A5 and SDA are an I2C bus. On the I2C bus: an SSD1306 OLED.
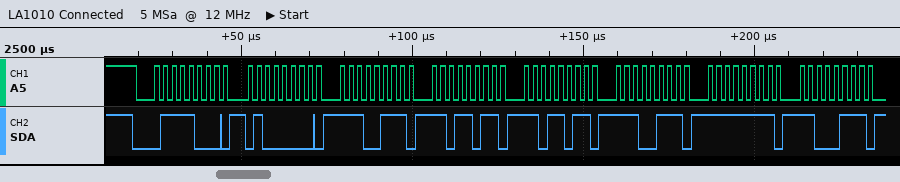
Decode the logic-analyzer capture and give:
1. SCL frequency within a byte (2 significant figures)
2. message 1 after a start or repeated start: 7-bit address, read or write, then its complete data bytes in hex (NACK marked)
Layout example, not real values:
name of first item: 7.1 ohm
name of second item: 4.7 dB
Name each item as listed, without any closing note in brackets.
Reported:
SCL frequency within a byte: 400 kHz
message 1 after a start or repeated start: 7-bit address, read or write, then its complete data bytes in hex: 0x3C write: 40 E7 DB DB E7 FF C7
